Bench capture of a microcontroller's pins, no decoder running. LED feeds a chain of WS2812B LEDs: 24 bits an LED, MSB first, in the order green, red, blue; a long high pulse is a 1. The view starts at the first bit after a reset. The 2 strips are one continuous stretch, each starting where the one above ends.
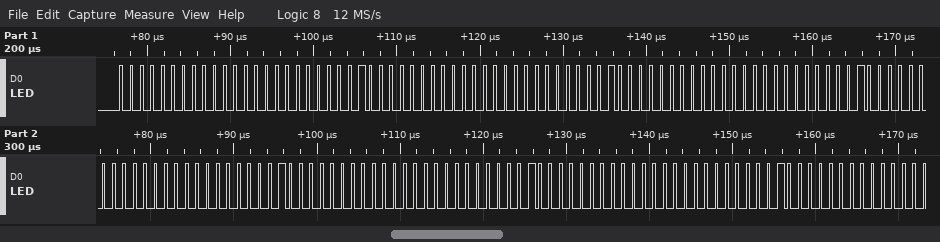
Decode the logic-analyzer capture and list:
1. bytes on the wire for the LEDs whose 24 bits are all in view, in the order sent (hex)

00 00 01 00 00 01 00 00 01 00 00 01 00 00 01 00 00 01
